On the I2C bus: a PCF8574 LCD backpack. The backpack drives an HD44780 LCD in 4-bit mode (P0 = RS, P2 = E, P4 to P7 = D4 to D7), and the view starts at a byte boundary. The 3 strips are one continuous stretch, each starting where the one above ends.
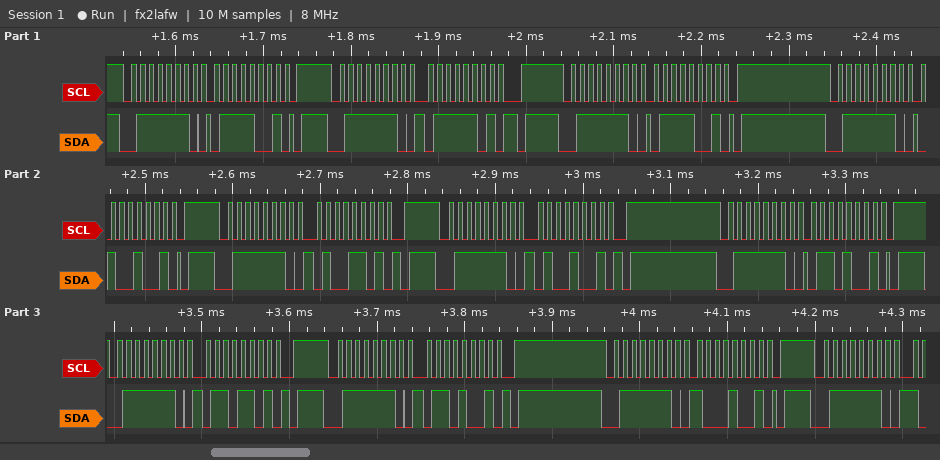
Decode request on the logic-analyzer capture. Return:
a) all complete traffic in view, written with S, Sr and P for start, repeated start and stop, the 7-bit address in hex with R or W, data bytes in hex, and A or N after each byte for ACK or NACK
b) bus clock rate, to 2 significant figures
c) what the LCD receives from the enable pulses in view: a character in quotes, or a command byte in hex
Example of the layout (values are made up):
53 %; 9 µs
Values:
S 3FW A 79 A P S 3FW A 7D A P S 3FW A 79 A P S 3FW A 49 A P S 3FW A 4D A P S 3FW A 49 A P S 3FW A 69 A P S 3FW A 6D A P S 3FW A 69 A P S 3FW A 89 A P S 3FW A; 100 kHz; 't'
